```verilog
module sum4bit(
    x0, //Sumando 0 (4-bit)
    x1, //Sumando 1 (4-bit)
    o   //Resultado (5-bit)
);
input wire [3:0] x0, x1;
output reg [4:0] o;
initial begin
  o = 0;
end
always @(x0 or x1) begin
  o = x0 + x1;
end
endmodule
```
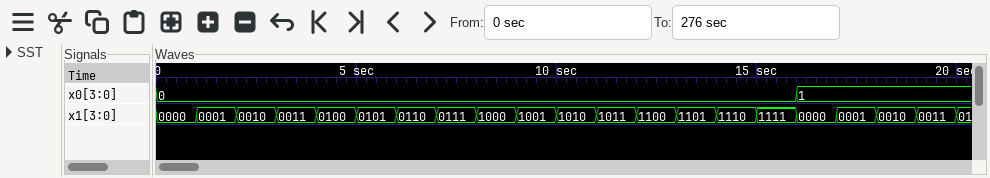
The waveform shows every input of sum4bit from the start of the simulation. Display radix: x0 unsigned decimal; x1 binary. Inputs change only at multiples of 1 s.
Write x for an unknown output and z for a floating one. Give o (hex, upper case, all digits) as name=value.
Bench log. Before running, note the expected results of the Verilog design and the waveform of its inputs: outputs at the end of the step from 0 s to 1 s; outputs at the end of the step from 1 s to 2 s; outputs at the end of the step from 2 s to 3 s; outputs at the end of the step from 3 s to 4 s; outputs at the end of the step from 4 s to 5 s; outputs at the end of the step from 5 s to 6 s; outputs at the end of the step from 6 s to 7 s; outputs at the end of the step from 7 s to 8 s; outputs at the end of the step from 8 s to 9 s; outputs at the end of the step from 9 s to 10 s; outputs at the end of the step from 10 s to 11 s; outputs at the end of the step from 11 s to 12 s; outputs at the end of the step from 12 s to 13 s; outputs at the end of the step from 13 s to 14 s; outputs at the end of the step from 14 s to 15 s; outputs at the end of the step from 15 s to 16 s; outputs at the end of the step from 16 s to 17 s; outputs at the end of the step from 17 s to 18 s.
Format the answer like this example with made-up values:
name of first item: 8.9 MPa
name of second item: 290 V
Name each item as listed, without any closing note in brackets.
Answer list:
outputs at the end of the step from 0 s to 1 s: o=00
outputs at the end of the step from 1 s to 2 s: o=01
outputs at the end of the step from 2 s to 3 s: o=02
outputs at the end of the step from 3 s to 4 s: o=03
outputs at the end of the step from 4 s to 5 s: o=04
outputs at the end of the step from 5 s to 6 s: o=05
outputs at the end of the step from 6 s to 7 s: o=06
outputs at the end of the step from 7 s to 8 s: o=07
outputs at the end of the step from 8 s to 9 s: o=08
outputs at the end of the step from 9 s to 10 s: o=09
outputs at the end of the step from 10 s to 11 s: o=0A
outputs at the end of the step from 11 s to 12 s: o=0B
outputs at the end of the step from 12 s to 13 s: o=0C
outputs at the end of the step from 13 s to 14 s: o=0D
outputs at the end of the step from 14 s to 15 s: o=0E
outputs at the end of the step from 15 s to 16 s: o=0F
outputs at the end of the step from 16 s to 17 s: o=01
outputs at the end of the step from 17 s to 18 s: o=02
